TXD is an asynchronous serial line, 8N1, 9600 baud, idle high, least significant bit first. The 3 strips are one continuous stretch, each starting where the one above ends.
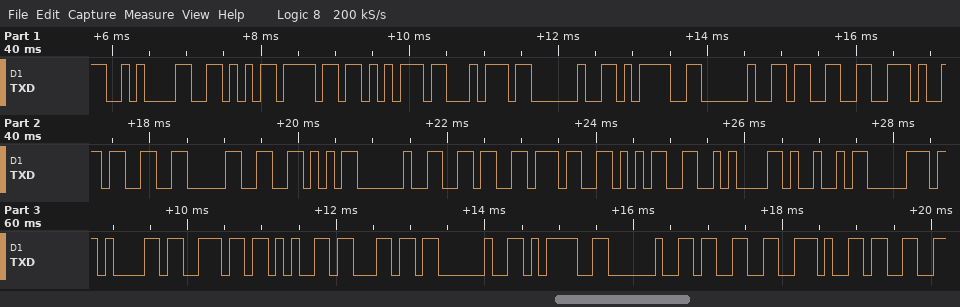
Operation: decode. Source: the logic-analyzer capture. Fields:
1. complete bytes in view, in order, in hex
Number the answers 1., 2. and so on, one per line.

1. 0A 56 6F 75 74 20 3D 20 33 2E 33 30 56 20 36 37 35 0A 49 70 61 6E 65 6C 20 3D 20 33 2E 33
